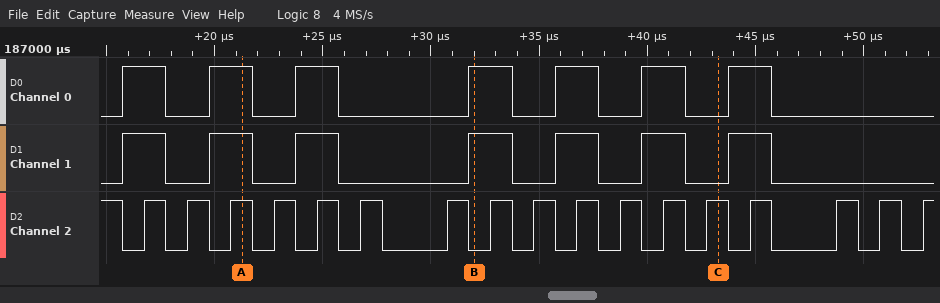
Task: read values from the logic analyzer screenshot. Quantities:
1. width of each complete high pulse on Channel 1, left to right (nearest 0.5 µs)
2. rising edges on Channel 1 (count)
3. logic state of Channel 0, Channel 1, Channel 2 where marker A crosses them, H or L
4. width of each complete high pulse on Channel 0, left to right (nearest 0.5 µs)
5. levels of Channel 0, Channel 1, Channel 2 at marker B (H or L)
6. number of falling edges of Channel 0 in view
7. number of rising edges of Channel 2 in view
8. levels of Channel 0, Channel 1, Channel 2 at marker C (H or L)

2 µs, 2 µs, 2 µs, 2 µs, 2 µs, 2 µs, 2 µs
7
Channel 0=H, Channel 1=H, Channel 2=H
2 µs, 2 µs, 2 µs, 2 µs, 2 µs, 2 µs, 2 µs
Channel 0=H, Channel 1=H, Channel 2=L
7
17
Channel 0=L, Channel 1=L, Channel 2=H
